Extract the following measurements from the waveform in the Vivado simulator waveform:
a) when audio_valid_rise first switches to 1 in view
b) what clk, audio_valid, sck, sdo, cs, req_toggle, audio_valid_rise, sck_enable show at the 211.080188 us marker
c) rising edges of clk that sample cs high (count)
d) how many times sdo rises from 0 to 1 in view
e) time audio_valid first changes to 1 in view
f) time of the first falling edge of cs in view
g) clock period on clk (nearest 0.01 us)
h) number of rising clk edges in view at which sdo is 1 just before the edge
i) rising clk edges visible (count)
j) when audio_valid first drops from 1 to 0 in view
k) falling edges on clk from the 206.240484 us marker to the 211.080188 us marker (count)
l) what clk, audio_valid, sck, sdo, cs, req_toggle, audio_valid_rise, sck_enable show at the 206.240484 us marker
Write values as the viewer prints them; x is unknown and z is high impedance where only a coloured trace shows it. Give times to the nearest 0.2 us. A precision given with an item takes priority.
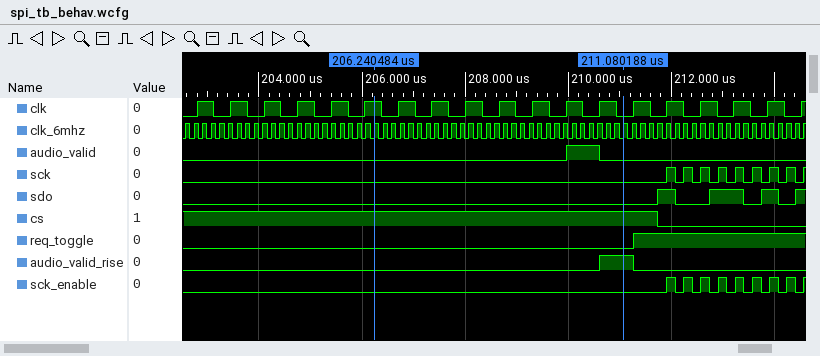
210.6 us
clk=0, audio_valid=0, sck=0, sdo=0, cs=1, req_toggle=0, audio_valid_rise=1, sck_enable=0
14
4
210 us
211.8 us
0.65 us
4
19
210.6 us
8
clk=1, audio_valid=0, sck=0, sdo=0, cs=1, req_toggle=0, audio_valid_rise=0, sck_enable=0
